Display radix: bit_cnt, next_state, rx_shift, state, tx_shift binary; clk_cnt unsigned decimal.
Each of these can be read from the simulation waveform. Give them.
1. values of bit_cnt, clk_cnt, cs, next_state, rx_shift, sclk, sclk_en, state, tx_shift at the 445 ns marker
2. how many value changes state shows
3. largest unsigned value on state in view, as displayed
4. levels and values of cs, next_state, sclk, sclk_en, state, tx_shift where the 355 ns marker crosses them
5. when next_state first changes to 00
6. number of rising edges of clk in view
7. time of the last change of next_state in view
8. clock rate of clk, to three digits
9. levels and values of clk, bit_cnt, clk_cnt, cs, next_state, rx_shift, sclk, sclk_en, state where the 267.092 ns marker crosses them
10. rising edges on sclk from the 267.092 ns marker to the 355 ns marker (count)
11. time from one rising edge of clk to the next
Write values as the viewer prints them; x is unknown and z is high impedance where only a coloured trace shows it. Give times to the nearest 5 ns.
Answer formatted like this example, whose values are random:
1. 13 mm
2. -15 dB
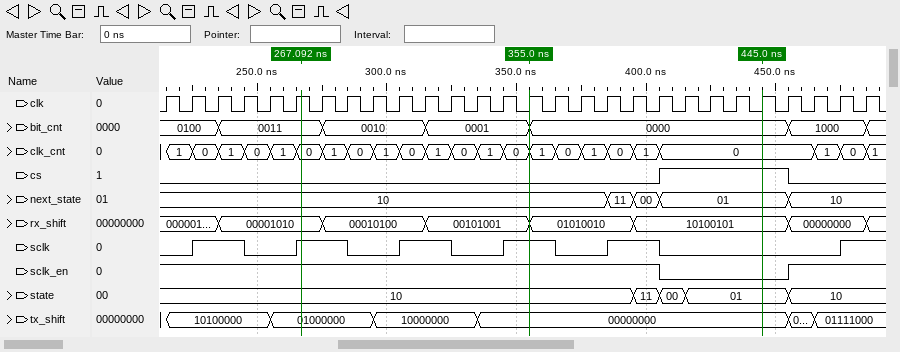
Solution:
1. bit_cnt=0000, clk_cnt=0, cs=1, next_state=01, rx_shift=10100101, sclk=0, sclk_en=0, state=01, tx_shift=00000000
2. 4
3. 11
4. cs=0, next_state=10, sclk=1, sclk_en=1, state=10, tx_shift=00000000
5. 395 ns
6. 28
7. 455 ns
8. 100 MHz
9. clk=1, bit_cnt=0011, clk_cnt=0, cs=0, next_state=10, rx_shift=00001010, sclk=1, sclk_en=1, state=10
10. 2
11. 10 ns
